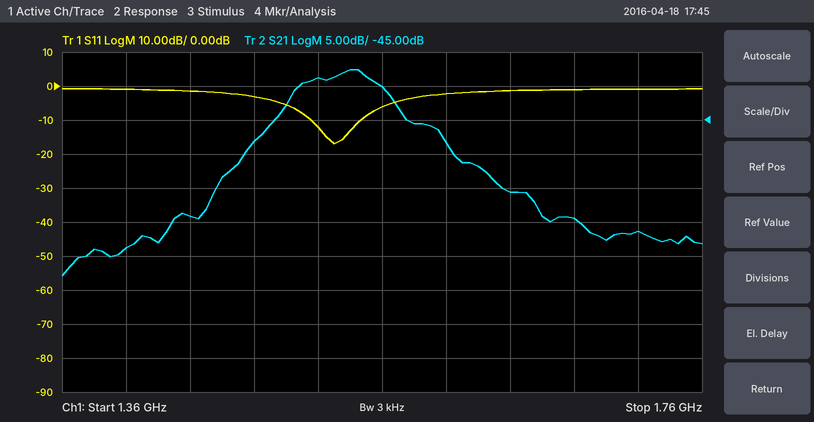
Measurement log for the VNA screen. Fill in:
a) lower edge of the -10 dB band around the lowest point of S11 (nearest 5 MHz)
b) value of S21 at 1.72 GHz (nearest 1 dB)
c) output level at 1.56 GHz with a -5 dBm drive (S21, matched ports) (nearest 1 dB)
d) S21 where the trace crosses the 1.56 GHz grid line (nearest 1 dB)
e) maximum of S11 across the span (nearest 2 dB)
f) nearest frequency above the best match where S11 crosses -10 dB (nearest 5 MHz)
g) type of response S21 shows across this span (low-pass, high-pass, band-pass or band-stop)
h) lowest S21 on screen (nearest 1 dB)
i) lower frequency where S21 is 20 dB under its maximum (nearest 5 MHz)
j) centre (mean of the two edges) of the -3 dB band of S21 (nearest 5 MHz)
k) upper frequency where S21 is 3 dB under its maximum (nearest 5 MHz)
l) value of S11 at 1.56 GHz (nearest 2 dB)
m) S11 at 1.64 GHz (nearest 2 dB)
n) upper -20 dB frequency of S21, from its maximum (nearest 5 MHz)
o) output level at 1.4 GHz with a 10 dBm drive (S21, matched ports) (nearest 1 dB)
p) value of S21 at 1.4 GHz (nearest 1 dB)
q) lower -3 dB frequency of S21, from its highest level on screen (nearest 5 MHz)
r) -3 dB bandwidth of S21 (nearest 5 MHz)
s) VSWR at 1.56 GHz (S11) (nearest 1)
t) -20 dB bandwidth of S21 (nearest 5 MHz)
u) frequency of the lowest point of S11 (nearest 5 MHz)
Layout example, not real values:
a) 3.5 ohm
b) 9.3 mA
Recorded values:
a) 1.515 GHz
b) -61 dB
c) -45 dBm
d) -40 dB
e) 0 dB
f) 1.545 GHz
g) band-pass
h) -68 dB
i) 1.450 GHz
j) 1.535 GHz
k) 1.560 GHz
l) -6 dB
m) -2 dB
n) 1.655 GHz
o) -54 dBm
p) -64 dB
q) 1.505 GHz
r) 55 MHz
s) 3
t) 205 MHz
u) 1.530 GHz
